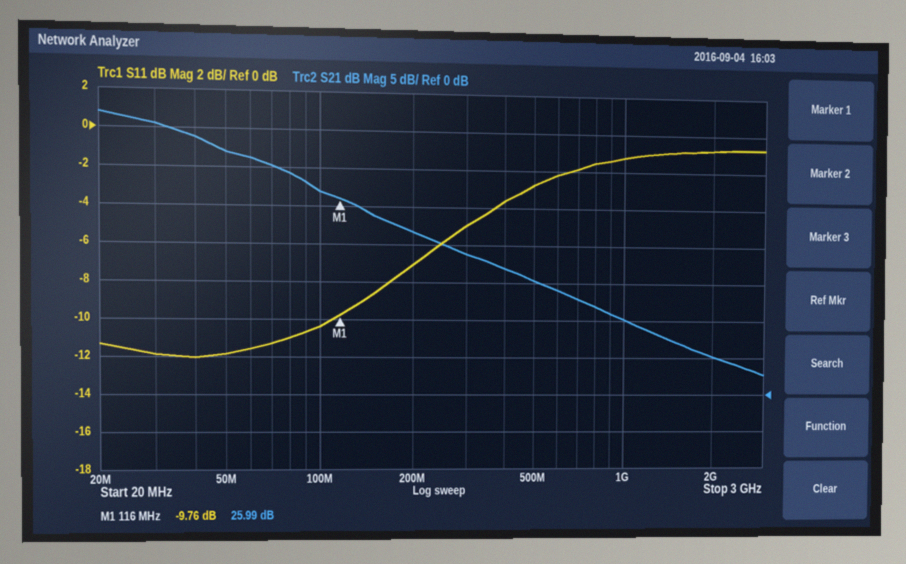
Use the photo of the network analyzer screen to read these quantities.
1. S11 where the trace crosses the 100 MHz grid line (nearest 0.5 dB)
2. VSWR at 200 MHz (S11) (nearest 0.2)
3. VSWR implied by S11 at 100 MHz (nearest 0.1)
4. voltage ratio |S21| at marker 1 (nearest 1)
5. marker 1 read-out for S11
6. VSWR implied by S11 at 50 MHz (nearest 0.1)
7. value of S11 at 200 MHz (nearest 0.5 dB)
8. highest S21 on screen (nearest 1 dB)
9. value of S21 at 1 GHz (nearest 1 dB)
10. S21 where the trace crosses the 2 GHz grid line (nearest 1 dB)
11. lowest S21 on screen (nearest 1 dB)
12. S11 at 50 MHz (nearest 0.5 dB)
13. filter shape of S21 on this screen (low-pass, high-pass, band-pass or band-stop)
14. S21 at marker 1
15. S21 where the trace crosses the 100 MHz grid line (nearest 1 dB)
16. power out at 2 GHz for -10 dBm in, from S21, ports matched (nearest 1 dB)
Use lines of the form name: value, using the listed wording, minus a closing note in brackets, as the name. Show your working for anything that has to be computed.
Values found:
S11 where the trace crosses the 100 MHz grid line: -10.5 dB
VSWR at 200 MHz (S11): |Γ| = 10^(-7/20) = 0.4467; VSWR = (1 + 0.4467)/(1 − 0.4467) ≈ 2.6
VSWR implied by S11 at 100 MHz: |Γ| = 10^(-10.5/20) = 0.2985; VSWR = (1 + 0.2985)/(1 − 0.2985) ≈ 1.9
voltage ratio |S21| at marker 1: 10^(25.99/20) ≈ 20
marker 1 read-out for S11: -9.76 dB
VSWR implied by S11 at 50 MHz: |Γ| = 10^(-12/20) = 0.2512; VSWR = (1 + 0.2512)/(1 − 0.2512) ≈ 1.7
value of S11 at 200 MHz: -7.0 dB
highest S21 on screen: 37 dB
value of S21 at 1 GHz: 10 dB
S21 where the trace crosses the 2 GHz grid line: 5 dB
lowest S21 on screen: 3 dB
S11 at 50 MHz: -12.0 dB
filter shape of S21 on this screen: low-pass
S21 at marker 1: 25.99 dB
S21 where the trace crosses the 100 MHz grid line: 27 dB
power out at 2 GHz for -10 dBm in, from S21, ports matched: -10 dBm + (5 dB) = -5 dBm
